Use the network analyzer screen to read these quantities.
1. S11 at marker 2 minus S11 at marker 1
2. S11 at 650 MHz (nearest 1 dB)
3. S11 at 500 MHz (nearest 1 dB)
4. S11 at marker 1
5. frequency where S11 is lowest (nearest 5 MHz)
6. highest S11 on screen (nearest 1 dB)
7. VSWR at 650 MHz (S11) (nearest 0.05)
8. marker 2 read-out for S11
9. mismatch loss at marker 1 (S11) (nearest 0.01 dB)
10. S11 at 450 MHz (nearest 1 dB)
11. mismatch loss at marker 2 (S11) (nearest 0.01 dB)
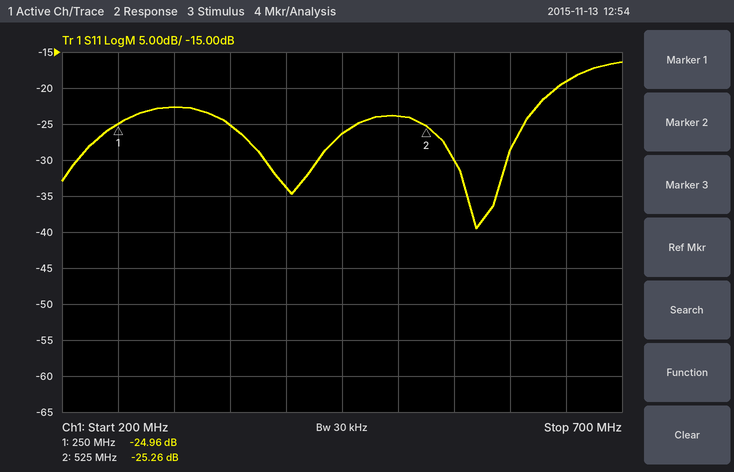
-0.30 dB
-19 dB
-24 dB
-24.96 dB
570 MHz
-16 dB
1.25
-25.26 dB
0.01 dB
-26 dB
0.01 dB
